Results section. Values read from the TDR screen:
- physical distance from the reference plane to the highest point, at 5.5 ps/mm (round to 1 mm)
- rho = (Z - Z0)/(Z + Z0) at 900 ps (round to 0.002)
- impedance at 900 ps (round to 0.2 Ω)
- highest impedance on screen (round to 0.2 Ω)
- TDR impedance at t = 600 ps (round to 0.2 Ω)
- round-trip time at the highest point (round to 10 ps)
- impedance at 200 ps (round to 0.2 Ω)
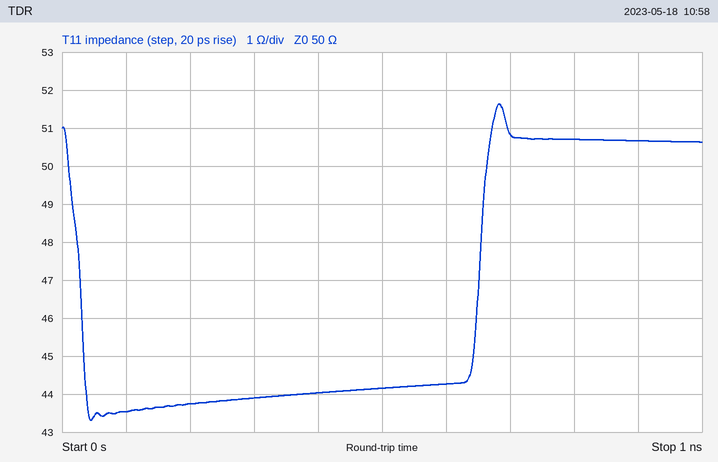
62 mm
+0.006
50.6 Ω
51.6 Ω
44.2 Ω
680 ps
43.8 Ω
